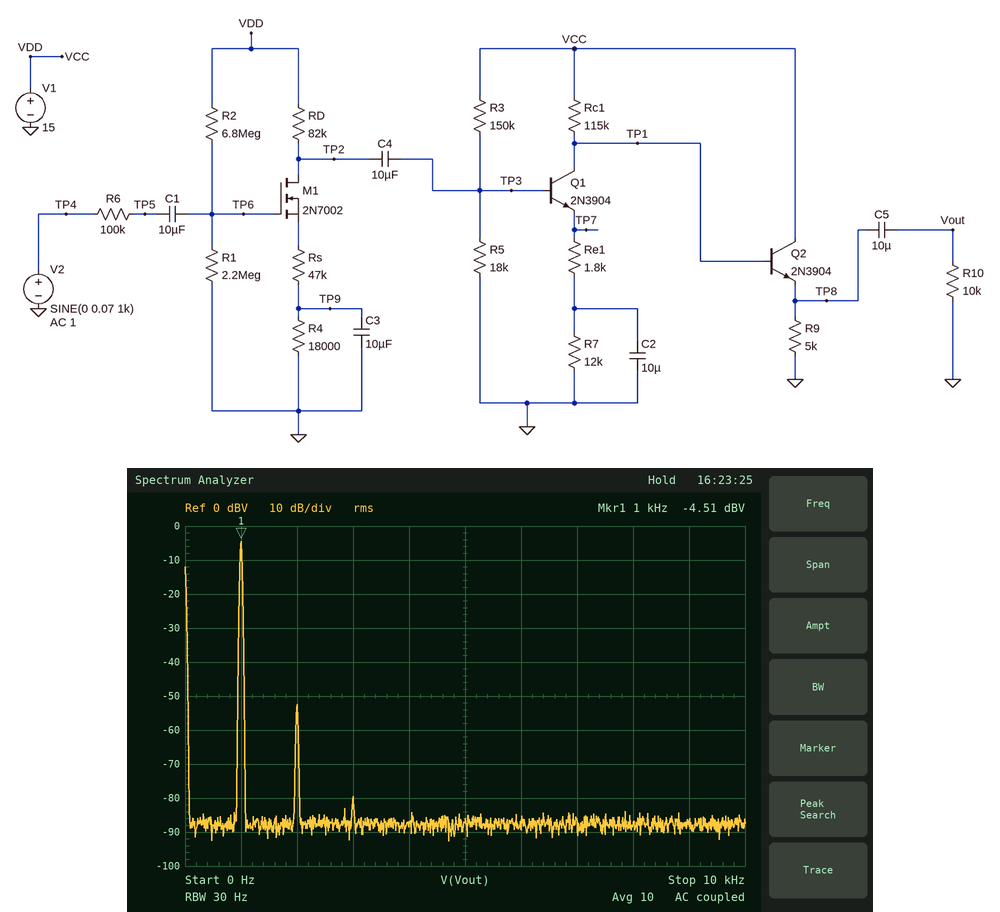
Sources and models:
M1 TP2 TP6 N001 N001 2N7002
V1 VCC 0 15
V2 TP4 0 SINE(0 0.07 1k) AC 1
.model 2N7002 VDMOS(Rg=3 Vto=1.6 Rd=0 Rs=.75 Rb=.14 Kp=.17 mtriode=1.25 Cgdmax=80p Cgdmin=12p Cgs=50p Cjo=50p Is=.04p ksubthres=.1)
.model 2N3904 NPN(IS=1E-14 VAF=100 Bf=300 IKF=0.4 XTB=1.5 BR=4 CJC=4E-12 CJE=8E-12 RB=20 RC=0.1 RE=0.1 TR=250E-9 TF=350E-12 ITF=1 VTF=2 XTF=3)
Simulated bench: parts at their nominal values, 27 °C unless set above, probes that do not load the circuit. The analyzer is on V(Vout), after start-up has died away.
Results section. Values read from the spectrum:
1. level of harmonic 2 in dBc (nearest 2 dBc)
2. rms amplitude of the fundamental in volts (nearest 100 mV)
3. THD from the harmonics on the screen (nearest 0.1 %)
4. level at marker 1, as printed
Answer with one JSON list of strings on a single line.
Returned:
["-48 dBc", "600 mV", "0.4 %", "-4.51 dBV"]
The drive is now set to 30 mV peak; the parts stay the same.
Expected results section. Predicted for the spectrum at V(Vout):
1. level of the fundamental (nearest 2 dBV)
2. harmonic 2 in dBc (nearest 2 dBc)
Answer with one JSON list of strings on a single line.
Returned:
["-12 dBV", "-56 dBc"]
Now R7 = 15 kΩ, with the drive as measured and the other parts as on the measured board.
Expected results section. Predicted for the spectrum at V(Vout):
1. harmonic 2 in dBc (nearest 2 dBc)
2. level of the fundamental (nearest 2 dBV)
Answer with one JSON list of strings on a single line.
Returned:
["-44 dBc", "-4 dBV"]
